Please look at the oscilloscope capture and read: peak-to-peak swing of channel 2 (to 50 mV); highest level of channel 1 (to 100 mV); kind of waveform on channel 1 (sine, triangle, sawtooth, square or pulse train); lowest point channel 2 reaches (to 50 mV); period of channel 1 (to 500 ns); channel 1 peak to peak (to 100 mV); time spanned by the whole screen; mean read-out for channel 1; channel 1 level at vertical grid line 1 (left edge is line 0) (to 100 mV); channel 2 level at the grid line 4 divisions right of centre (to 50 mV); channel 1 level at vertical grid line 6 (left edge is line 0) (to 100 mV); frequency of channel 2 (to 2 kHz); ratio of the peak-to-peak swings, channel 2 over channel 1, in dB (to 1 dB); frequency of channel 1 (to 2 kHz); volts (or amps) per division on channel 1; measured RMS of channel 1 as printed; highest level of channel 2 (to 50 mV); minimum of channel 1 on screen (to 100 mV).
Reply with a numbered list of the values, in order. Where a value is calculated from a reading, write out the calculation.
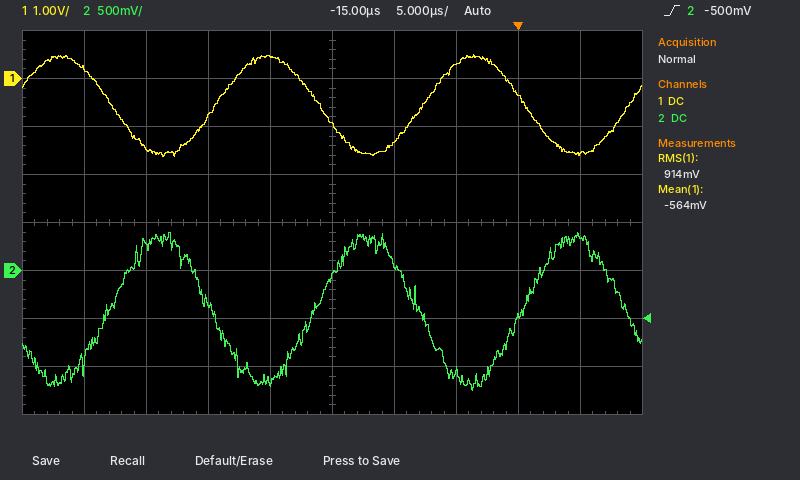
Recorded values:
1. 400 mV − (-1.25 V) = 1.65 V
2. 500 mV
3. sine
4. -1.25 V
5. 16.5 µs
6. 500 mV − (-1.6 V) = 2.1 V
7. 50 µs
8. -564 mV
9. 200 mV
10. 350 mV
11. -1.3 V
12. 60 kHz
13. 20 log10(1.65 V / 2.1 V) ≈ -2 dB
14. 1 / 16.5 µs ≈ 60.6 kHz, so 60 kHz to the nearest 2 kHz
15. 1 V
16. 914 mV
17. 400 mV
18. -1.6 V
